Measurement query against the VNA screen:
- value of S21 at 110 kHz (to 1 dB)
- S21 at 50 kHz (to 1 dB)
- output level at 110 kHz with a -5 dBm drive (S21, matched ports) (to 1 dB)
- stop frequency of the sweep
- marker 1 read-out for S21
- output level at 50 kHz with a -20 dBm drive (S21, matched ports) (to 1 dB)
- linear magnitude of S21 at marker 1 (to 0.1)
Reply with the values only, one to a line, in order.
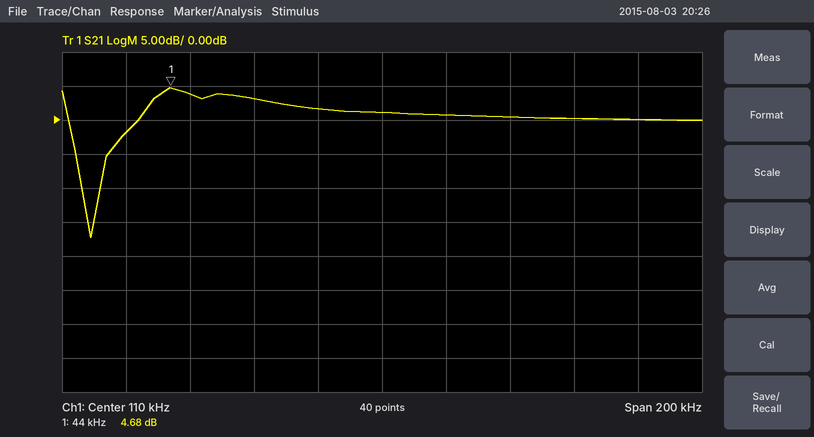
1 dB
4 dB
-4 dBm
210 kHz
4.68 dB
-16 dBm
1.7
